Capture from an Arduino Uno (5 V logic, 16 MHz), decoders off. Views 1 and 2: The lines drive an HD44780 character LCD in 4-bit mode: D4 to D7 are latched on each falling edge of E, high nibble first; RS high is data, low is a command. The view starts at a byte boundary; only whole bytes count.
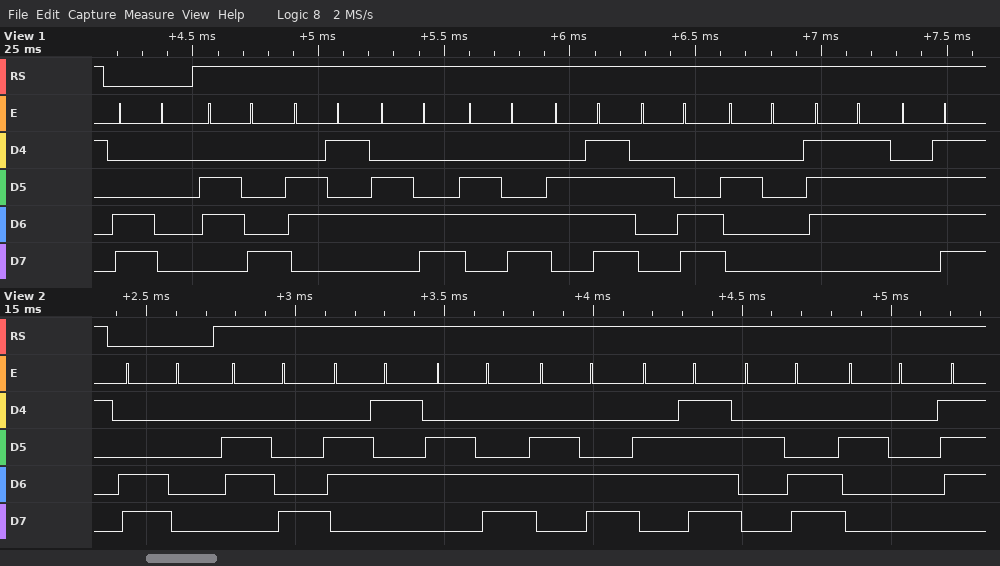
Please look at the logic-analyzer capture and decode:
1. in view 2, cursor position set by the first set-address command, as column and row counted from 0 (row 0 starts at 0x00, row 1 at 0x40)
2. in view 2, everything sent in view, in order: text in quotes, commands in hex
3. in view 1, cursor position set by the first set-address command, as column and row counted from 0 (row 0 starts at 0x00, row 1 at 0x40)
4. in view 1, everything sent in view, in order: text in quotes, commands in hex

column 0, row 1
0xC0 "hello, "
column 0, row 1
0xC0 "hello, wo"
